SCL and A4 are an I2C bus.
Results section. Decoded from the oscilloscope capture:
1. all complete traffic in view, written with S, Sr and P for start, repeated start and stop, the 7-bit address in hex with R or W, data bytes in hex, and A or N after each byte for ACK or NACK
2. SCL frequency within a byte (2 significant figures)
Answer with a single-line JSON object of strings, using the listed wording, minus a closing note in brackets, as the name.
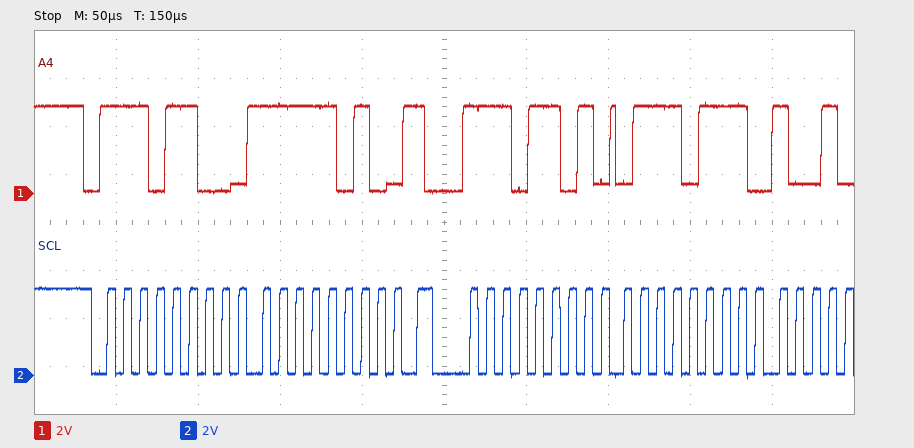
{"all complete traffic in view, written with S, Sr and P for start, repeated start and stop, the 7-bit address in hex with R or W, data bytes in hex, and A or N after each byte for ACK or NACK": "S 76W A FA A Sr 76R A 77 A", "SCL frequency within a byte": "100 kHz"}
